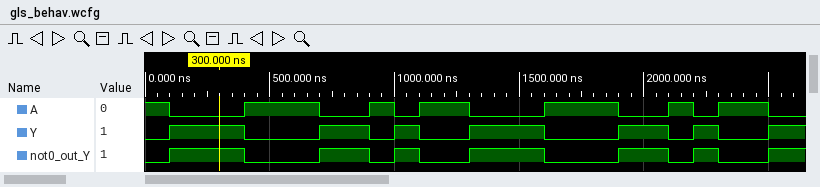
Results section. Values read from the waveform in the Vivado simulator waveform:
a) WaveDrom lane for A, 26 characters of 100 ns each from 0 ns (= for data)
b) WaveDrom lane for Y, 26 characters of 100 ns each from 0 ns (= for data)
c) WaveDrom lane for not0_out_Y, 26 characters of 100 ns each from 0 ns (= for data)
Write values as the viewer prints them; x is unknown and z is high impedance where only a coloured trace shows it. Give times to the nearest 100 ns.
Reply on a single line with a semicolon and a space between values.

{name: 'A', wave: '10..1..0.101.0..1..0.101.0'}; {name: 'Y', wave: '01..0..1.010.1..0..1.010.1'}; {name: 'not0_out_Y', wave: '01..0..1.010.1..0..1.010.1'}
